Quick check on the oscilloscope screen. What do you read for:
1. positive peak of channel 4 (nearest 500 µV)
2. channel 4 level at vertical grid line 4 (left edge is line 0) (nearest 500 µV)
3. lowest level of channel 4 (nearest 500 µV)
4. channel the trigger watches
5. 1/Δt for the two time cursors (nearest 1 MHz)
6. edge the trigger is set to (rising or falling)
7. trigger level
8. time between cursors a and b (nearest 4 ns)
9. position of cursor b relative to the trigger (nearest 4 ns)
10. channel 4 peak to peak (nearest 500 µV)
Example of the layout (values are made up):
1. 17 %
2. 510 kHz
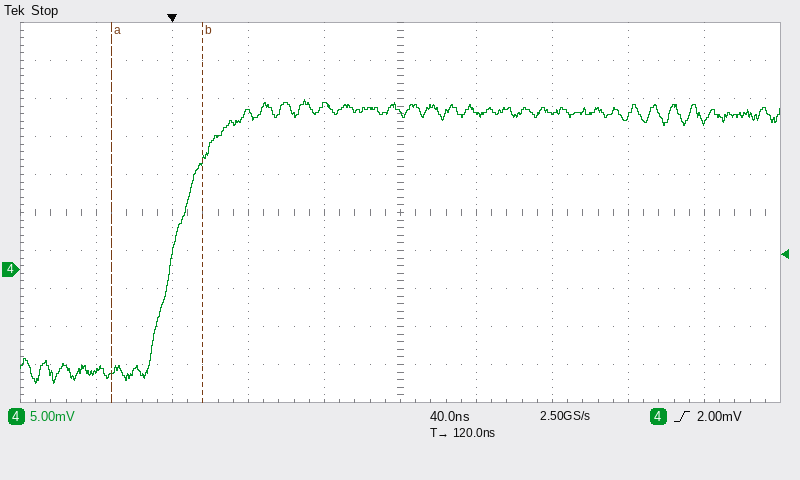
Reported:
1. 22.5 mV
2. 21.5 mV
3. -15.0 mV
4. channel 4
5. 21 MHz
6. rising
7. 2.00 mV
8. 48 ns
9. +16 ns
10. 37.5 mV
